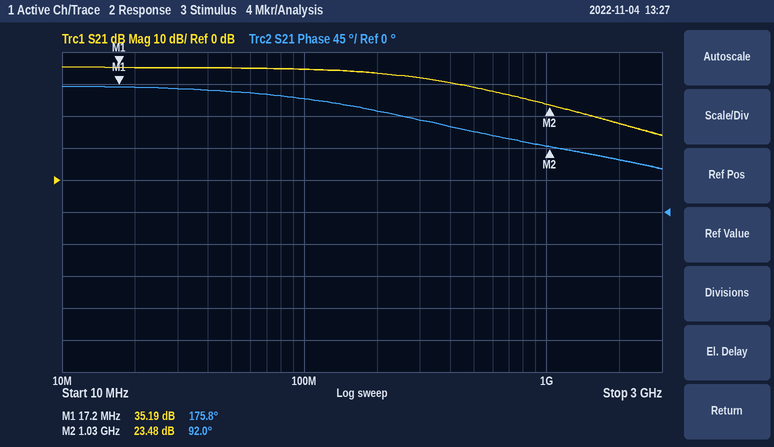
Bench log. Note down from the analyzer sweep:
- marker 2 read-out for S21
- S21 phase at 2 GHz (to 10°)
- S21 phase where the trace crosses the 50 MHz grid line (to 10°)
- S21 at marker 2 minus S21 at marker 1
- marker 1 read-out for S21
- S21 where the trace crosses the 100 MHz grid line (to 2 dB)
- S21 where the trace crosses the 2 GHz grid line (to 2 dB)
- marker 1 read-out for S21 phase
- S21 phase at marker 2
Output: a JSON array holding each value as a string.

["23.48 dB", "70°", "170°", "-11.71 dB", "35.19 dB", "34 dB", "18 dB", "175.8°", "92.0°"]
